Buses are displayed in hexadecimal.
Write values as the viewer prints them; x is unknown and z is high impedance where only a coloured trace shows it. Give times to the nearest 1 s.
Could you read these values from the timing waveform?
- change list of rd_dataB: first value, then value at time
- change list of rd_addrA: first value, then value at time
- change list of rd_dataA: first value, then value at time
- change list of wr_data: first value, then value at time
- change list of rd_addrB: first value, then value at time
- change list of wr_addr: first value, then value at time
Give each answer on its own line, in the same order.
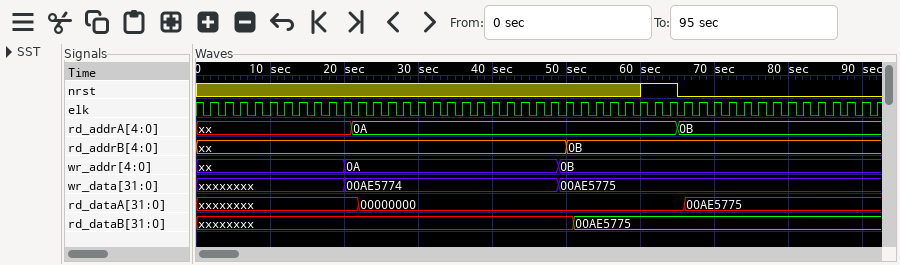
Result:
xxxxxxxx, 00AE5775 at 51 s
xx, 0A at 21 s, 0B at 65 s
xxxxxxxx, 00000000 at 22 s, 00AE5775 at 66 s
xxxxxxxx, 00AE5774 at 20 s, 00AE5775 at 49 s
xx, 0B at 50 s
xx, 0A at 20 s, 0B at 49 s
